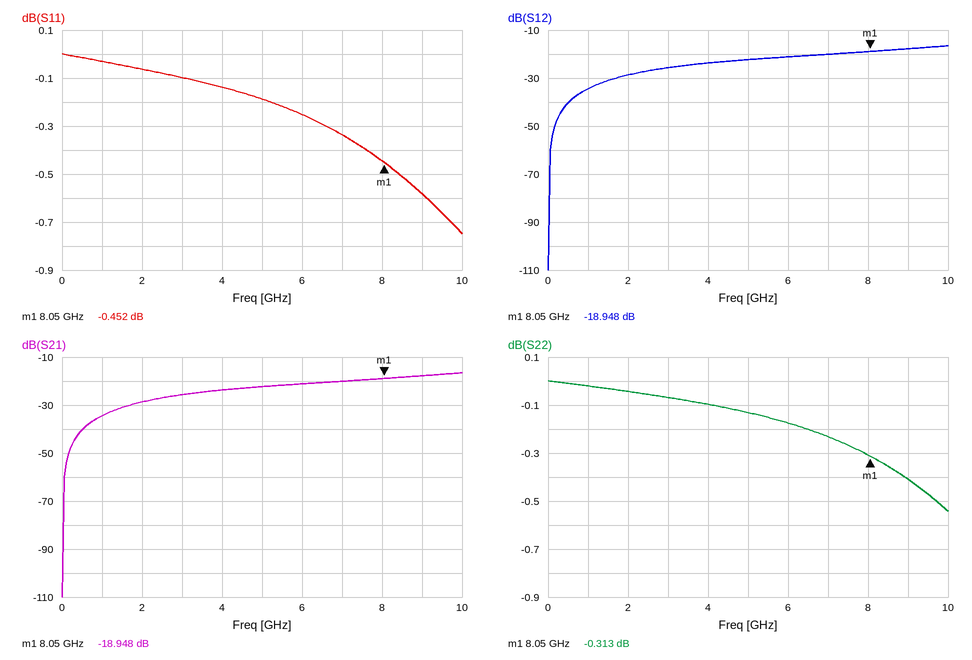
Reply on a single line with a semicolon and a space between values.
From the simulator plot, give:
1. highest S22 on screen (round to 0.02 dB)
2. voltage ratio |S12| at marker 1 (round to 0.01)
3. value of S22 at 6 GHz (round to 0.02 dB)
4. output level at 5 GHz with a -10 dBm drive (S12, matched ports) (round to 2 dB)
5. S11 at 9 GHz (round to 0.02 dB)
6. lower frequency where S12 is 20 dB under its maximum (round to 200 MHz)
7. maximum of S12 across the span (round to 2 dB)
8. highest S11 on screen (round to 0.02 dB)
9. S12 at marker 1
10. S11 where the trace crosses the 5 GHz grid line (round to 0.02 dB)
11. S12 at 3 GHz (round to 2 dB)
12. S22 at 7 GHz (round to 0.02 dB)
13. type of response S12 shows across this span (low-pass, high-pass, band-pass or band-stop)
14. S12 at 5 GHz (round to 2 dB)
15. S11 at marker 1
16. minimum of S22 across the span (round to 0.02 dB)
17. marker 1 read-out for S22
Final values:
0.00 dB; 0.11; -0.18 dB; -32 dBm; -0.58 dB; 800 MHz; -16 dB; 0.00 dB; -18.948 dB; -0.18 dB; -26 dB; -0.24 dB; high-pass; -22 dB; -0.452 dB; -0.54 dB; -0.313 dB
